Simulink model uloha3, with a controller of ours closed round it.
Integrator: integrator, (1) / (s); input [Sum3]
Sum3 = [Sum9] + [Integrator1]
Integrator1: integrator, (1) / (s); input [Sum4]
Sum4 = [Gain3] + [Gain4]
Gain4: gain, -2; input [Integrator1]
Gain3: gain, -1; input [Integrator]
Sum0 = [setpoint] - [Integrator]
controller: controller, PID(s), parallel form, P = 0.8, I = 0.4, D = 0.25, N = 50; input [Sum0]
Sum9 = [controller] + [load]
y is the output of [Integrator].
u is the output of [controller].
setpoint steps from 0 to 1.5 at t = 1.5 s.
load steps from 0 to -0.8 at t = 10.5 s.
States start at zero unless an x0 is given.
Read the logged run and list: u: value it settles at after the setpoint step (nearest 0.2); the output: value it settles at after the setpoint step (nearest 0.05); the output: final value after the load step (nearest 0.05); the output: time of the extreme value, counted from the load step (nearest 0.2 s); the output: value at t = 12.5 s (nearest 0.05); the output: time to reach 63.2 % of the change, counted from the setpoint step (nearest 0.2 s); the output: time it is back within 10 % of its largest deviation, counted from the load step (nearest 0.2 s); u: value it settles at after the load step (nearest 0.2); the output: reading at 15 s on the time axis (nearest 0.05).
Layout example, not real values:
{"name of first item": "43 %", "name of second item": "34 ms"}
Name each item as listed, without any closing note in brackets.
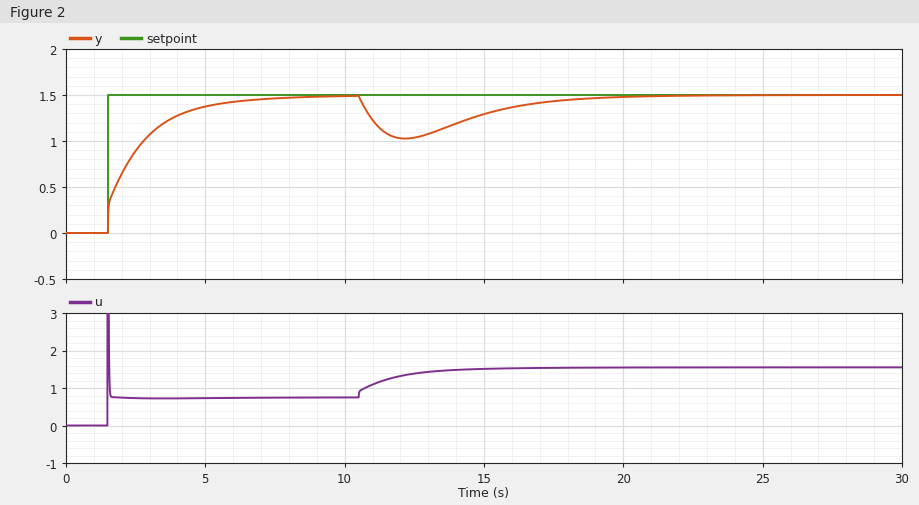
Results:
{"u: value it settles at after the setpoint step": "0.8", "the output: value it settles at after the setpoint step": "1.50", "the output: final value after the load step": "1.50", "the output: time of the extreme value, counted from the load step": "1.6 s", "the output: value at t = 12.5 s": "1.05", "the output: time to reach 63.2 % of the change, counted from the setpoint step": "1.2 s", "the output: time it is back within 10 % of its largest deviation, counted from the load step": "7.8 s", "u: value it settles at after the load step": "1.6", "the output: reading at 15 s on the time axis": "1.30"}
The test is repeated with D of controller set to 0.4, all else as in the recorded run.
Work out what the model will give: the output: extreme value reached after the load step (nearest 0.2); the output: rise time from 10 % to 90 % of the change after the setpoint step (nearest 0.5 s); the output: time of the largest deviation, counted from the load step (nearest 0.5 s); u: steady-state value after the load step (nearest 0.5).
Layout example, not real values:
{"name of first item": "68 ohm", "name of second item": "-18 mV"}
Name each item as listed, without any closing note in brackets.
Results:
{"the output: extreme value reached after the load step": "1.0", "the output: rise time from 10 % to 90 % of the change after the setpoint step": "3.5 s", "the output: time of the largest deviation, counted from the load step": "2.0 s", "u: steady-state value after the load step": "1.5"}
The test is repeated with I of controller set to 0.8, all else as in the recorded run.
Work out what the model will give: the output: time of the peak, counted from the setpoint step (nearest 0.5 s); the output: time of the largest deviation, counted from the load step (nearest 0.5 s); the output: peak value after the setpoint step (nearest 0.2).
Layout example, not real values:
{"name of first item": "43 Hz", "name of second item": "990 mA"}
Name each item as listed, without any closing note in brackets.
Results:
{"the output: time of the peak, counted from the setpoint step": "3.5 s", "the output: time of the largest deviation, counted from the load step": "1.5 s", "the output: peak value after the setpoint step": "1.6"}
